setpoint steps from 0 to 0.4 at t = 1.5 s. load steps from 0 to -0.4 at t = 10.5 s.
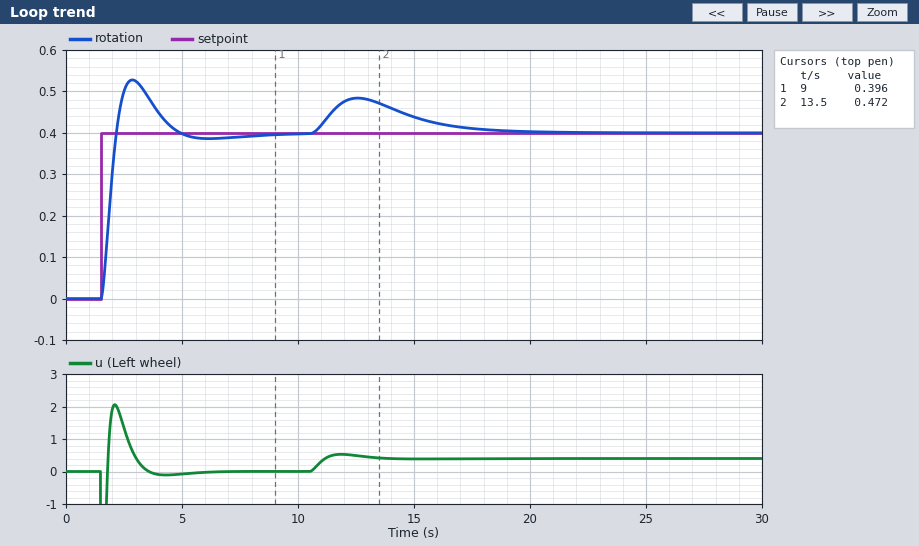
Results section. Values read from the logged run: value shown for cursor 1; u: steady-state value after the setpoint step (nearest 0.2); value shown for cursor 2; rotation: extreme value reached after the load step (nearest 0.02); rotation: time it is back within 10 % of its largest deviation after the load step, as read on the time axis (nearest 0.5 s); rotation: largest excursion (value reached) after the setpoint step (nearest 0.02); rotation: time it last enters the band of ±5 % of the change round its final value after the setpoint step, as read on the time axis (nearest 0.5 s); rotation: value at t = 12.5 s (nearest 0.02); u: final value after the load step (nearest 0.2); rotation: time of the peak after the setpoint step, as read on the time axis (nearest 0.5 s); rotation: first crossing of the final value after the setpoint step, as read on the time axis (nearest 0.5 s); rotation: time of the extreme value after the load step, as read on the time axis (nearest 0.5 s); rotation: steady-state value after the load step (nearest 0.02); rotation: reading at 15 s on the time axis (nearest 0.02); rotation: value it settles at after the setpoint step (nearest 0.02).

0.396
0.0
0.472
0.48
18.0 s
0.52
4.5 s
0.48
0.4
3.0 s
2.0 s
12.5 s
0.40
0.44
0.40
